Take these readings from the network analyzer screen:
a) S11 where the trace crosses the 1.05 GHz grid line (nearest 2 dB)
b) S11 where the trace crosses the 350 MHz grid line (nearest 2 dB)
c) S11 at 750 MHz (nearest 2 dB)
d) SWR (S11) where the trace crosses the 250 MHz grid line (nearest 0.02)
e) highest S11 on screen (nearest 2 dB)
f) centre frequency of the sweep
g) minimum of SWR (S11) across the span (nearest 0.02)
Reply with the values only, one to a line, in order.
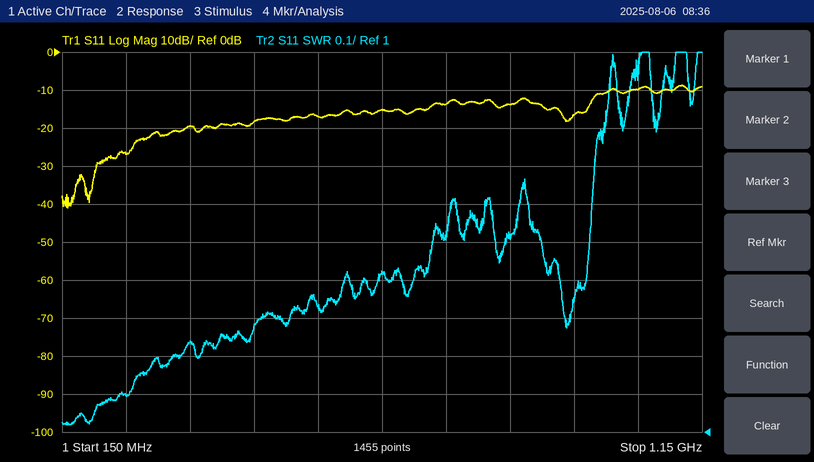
-10 dB
-20 dB
-14 dB
1.10
-8 dB
650 MHz
1.02
